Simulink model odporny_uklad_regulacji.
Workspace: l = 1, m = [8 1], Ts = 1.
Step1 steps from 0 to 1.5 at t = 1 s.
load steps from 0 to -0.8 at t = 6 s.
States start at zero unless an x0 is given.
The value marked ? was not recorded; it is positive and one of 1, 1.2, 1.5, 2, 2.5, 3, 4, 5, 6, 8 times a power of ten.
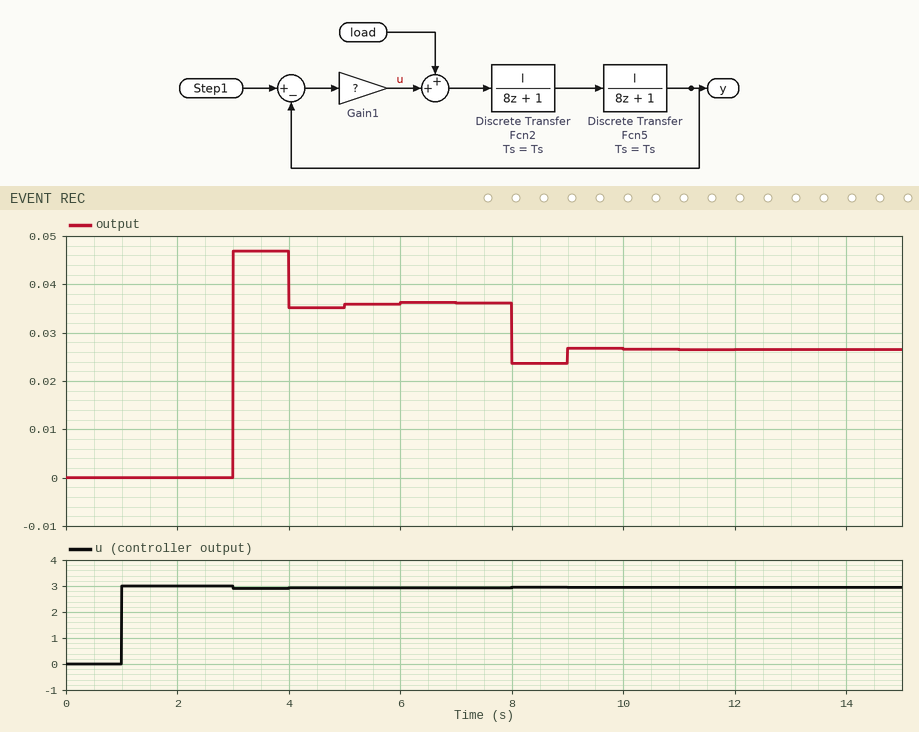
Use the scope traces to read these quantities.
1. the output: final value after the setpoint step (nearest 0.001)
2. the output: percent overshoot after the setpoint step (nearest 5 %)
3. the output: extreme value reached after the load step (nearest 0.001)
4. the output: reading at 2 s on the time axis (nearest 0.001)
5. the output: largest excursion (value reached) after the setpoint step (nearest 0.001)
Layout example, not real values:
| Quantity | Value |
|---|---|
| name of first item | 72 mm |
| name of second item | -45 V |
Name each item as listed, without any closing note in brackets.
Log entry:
| Quantity | Value |
|---|---|
| the output: final value after the setpoint step | 0.036 |
| the output: percent overshoot after the setpoint step | 30 % |
| the output: extreme value reached after the load step | 0.024 |
| the output: reading at 2 s on the time axis | 0.000 |
| the output: largest excursion (value reached) after the setpoint step | 0.047 |
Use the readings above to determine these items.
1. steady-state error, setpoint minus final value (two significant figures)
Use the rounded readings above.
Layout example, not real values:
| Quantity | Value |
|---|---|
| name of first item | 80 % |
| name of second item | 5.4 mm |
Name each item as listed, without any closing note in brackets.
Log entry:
| Quantity | Value |
|---|---|
| steady-state error, setpoint minus final value | 1.5 |
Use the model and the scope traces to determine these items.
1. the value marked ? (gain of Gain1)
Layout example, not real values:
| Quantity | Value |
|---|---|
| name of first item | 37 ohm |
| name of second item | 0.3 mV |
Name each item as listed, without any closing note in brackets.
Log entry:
| Quantity | Value |
|---|---|
| the value marked ? | 2 |
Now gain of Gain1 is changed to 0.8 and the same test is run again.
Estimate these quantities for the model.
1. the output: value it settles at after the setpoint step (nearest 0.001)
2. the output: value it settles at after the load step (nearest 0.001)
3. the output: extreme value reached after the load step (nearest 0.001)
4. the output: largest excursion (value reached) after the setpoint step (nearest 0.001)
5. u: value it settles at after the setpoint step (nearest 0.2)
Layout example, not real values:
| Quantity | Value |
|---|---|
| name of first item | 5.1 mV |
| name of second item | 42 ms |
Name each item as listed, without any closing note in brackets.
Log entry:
| Quantity | Value |
|---|---|
| the output: value it settles at after the setpoint step | 0.015 |
| the output: value it settles at after the load step | 0.005 |
| the output: extreme value reached after the load step | 0.002 |
| the output: largest excursion (value reached) after the setpoint step | 0.019 |
| u: value it settles at after the setpoint step | 1.2 |
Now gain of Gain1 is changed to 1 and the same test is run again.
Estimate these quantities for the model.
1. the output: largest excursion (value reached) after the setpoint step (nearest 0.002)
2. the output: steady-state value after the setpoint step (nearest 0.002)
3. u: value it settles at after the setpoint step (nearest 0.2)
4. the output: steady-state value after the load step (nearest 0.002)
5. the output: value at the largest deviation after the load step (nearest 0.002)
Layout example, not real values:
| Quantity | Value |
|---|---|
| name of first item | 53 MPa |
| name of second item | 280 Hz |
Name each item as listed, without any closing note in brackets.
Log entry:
| Quantity | Value |
|---|---|
| the output: largest excursion (value reached) after the setpoint step | 0.024 |
| the output: steady-state value after the setpoint step | 0.018 |
| u: value it settles at after the setpoint step | 1.4 |
| the output: steady-state value after the load step | 0.008 |
| the output: value at the largest deviation after the load step | 0.006 |
